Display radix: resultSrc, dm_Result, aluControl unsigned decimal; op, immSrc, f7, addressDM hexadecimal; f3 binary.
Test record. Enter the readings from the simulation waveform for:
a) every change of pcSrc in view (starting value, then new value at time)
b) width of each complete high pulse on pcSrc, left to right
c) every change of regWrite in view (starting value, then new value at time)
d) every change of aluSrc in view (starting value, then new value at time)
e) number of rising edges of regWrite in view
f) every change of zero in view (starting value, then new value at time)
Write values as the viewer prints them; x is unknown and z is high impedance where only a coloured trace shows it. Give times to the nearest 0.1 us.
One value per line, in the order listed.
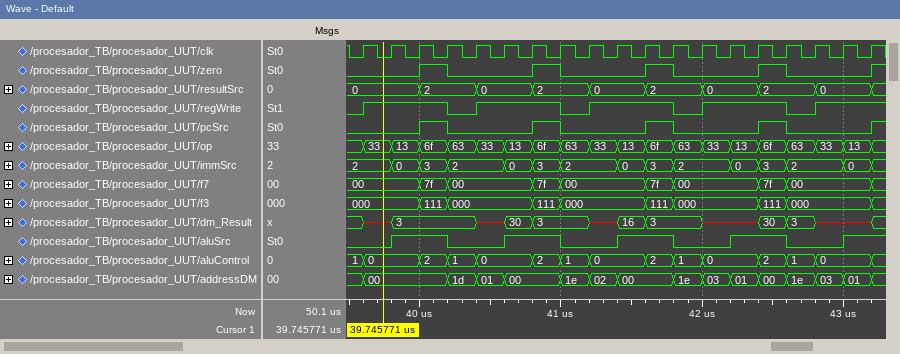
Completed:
0, 1 at 40 us, 0 at 40.2 us, 1 at 40.8 us, 0 at 41 us, 1 at 41.6 us, 0 at 41.8 us, 1 at 42.4 us, 0 at 42.6 us, 1 at 43.2 us
0.2 us, 0.2 us, 0.2 us, 0.2 us
0, 1 at 39.6 us, 0 at 40.2 us, 1 at 40.4 us, 0 at 41 us, 1 at 41.2 us, 0 at 41.8 us, 1 at 42 us, 0 at 42.6 us, 1 at 42.8 us
0, 1 at 39.8 us, 0 at 40.2 us, 1 at 40.6 us, 0 at 41 us, 1 at 41.4 us, 0 at 41.8 us, 1 at 42.2 us, 0 at 42.6 us, 1 at 43 us
5
0, 1 at 40 us, 0 at 40.2 us, 1 at 40.8 us, 0 at 41 us, 1 at 41.6 us, 0 at 41.8 us, 1 at 42.4 us, 0 at 42.6 us, 1 at 43.2 us
